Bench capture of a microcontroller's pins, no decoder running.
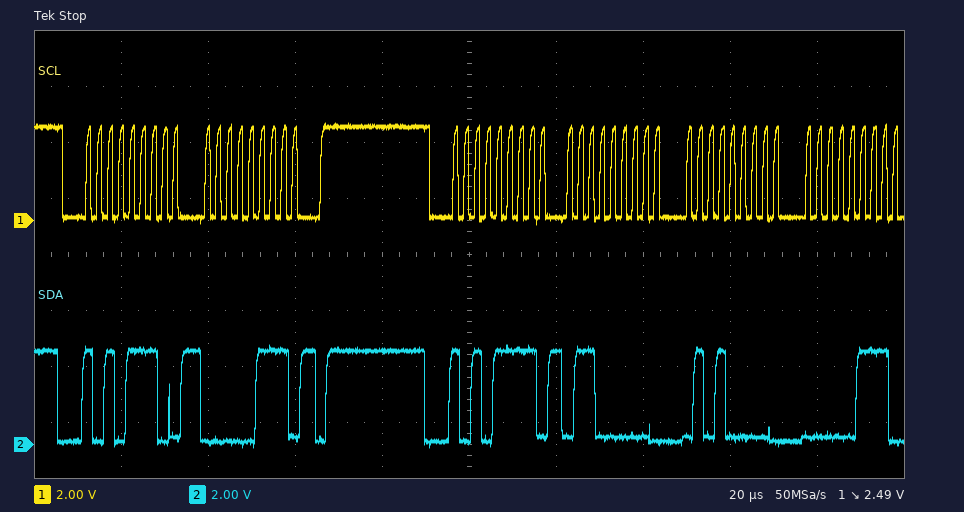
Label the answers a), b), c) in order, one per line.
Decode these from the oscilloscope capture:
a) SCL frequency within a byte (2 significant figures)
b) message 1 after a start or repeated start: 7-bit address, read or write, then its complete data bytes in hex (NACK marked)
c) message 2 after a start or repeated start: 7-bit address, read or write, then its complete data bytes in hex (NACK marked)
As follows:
a) 400 kHz
b) 0x57 write: 07
c) 0x57 read: 60 50 07
